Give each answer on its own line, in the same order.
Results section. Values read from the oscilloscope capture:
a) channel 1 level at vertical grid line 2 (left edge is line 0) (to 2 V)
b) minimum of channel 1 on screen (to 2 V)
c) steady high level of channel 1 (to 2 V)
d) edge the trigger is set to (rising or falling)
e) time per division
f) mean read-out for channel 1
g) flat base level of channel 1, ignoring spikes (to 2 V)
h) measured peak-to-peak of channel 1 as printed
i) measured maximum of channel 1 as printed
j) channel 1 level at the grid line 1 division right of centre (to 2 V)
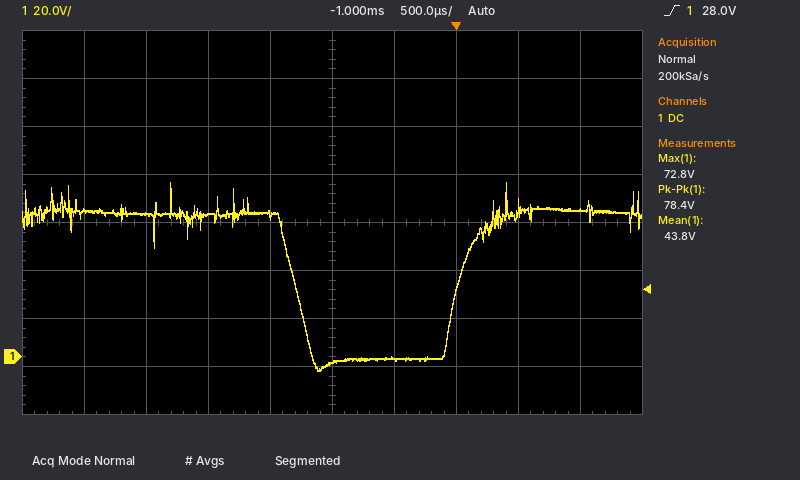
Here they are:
60 V
-6 V
60 V
rising
500 µs
43.8 V
0 V
78.4 V
72.8 V
0 V
